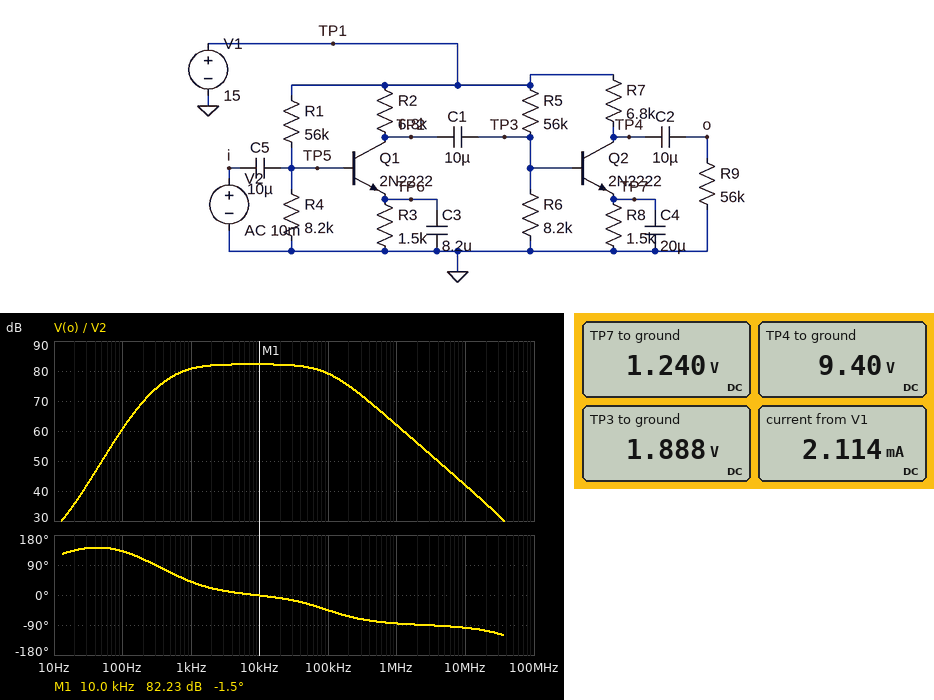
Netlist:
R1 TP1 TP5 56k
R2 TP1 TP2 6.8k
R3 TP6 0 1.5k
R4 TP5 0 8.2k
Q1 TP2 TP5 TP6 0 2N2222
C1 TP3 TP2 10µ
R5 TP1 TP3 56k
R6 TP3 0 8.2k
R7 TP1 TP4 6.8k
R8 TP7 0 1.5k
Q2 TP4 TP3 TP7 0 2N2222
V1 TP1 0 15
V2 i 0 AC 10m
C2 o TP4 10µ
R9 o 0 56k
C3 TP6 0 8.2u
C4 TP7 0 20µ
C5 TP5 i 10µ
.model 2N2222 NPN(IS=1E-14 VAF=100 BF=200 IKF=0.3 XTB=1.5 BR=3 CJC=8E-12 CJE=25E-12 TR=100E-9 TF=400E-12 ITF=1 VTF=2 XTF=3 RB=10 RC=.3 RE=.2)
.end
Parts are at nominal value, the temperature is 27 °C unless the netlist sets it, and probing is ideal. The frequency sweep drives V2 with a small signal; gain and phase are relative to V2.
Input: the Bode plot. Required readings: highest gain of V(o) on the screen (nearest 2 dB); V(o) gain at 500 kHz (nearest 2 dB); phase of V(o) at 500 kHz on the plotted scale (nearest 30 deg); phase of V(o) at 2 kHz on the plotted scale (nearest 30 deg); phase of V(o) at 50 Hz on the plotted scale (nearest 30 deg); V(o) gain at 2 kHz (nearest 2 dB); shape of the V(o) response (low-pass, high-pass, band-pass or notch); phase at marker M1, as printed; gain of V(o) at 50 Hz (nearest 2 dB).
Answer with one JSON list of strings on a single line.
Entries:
["82 dB", "68 dB", "-90 deg", "30 deg", "150 deg", "82 dB", "band-pass", "-1.5 deg", "50 dB"]
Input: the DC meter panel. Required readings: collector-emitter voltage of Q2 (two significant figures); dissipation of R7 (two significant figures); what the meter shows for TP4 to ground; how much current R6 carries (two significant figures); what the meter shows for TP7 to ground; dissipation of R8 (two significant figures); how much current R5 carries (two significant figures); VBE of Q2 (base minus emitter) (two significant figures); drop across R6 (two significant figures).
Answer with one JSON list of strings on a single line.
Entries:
["8.2 V", "4.6 mW", "9.40 V", "230 µA", "1.240 V", "1.0 mW", "230 µA", "650 mV", "1.9 V"]
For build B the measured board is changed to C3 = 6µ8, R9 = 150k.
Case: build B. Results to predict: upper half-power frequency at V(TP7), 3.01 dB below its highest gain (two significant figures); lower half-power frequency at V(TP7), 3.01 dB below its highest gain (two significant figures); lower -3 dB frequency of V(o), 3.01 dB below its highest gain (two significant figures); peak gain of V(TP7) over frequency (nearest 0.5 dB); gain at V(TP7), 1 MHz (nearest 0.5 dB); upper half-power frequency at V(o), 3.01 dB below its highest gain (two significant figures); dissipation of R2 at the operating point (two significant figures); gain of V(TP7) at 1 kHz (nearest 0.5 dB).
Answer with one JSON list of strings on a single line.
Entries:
["1.0 kHz", "120 Hz", "770 Hz", "25.5 dB", "-56.0 dB", "92 kHz", "4.6 mW", "22.5 dB"]
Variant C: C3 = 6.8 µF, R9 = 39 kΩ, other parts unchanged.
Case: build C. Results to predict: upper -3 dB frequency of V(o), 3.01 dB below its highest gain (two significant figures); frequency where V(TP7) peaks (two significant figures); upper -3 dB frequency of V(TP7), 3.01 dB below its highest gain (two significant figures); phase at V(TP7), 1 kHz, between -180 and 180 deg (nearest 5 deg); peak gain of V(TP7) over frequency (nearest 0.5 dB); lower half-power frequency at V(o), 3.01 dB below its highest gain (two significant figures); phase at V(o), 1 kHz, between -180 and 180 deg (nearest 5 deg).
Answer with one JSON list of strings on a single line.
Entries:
["100 kHz", "350 Hz", "1.0 kHz", "135 deg", "25.5 dB", "770 Hz", "45 deg"]
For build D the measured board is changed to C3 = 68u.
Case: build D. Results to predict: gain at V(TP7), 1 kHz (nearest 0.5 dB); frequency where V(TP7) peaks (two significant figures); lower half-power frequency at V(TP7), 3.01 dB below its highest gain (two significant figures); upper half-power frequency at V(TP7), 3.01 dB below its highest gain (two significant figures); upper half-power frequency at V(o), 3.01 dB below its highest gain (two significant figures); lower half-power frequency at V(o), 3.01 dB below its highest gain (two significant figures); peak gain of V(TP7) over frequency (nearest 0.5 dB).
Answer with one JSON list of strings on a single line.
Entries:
["24.5 dB", "110 Hz", "44 Hz", "290 Hz", "96 kHz", "190 Hz", "37.0 dB"]
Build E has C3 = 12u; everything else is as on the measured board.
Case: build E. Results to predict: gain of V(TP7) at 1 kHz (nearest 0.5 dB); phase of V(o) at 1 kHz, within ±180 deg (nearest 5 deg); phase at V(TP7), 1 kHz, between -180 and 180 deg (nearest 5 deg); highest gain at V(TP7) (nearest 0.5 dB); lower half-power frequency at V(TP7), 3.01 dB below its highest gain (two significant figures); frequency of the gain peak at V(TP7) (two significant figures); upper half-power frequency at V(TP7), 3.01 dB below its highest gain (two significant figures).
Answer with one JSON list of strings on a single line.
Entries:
["24.0 dB", "30 deg", "120 deg", "29.5 dB", "100 Hz", "260 Hz", "690 Hz"]
